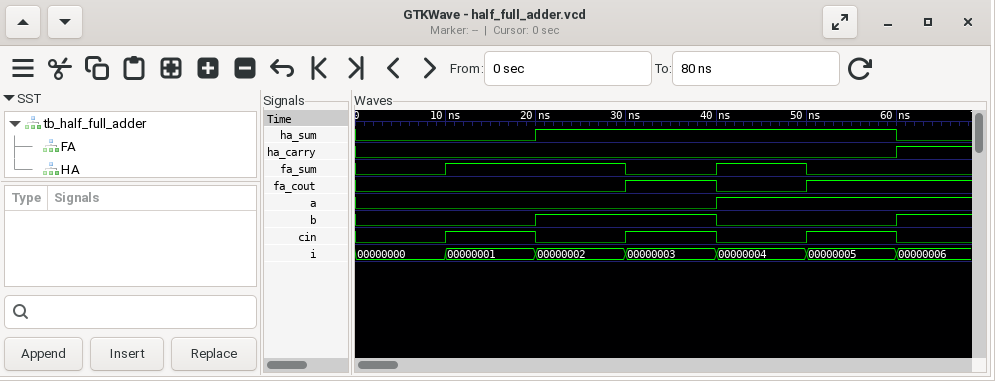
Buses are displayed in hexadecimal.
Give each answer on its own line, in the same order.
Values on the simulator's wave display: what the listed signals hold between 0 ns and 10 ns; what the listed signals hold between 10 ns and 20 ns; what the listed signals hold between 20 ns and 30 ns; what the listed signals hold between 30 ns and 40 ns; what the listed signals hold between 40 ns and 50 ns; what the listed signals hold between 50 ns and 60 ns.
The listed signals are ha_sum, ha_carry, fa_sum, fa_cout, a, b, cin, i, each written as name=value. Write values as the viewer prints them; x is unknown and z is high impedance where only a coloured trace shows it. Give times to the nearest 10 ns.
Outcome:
ha_sum=0, ha_carry=0, fa_sum=0, fa_cout=0, a=0, b=0, cin=0, i=00000000
ha_sum=0, ha_carry=0, fa_sum=1, fa_cout=0, a=0, b=0, cin=1, i=00000001
ha_sum=1, ha_carry=0, fa_sum=1, fa_cout=0, a=0, b=1, cin=0, i=00000002
ha_sum=1, ha_carry=0, fa_sum=0, fa_cout=1, a=0, b=1, cin=1, i=00000003
ha_sum=1, ha_carry=0, fa_sum=1, fa_cout=0, a=1, b=0, cin=0, i=00000004
ha_sum=1, ha_carry=0, fa_sum=0, fa_cout=1, a=1, b=0, cin=1, i=00000005
